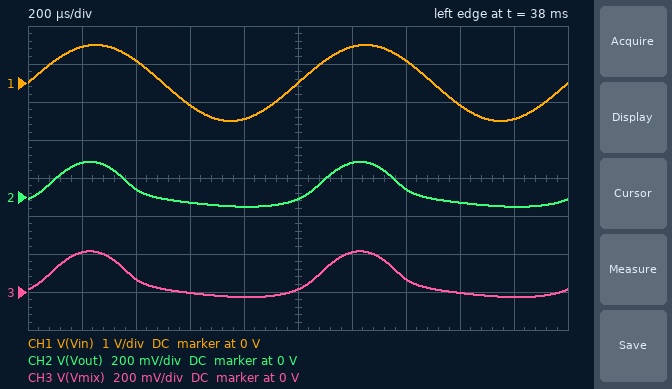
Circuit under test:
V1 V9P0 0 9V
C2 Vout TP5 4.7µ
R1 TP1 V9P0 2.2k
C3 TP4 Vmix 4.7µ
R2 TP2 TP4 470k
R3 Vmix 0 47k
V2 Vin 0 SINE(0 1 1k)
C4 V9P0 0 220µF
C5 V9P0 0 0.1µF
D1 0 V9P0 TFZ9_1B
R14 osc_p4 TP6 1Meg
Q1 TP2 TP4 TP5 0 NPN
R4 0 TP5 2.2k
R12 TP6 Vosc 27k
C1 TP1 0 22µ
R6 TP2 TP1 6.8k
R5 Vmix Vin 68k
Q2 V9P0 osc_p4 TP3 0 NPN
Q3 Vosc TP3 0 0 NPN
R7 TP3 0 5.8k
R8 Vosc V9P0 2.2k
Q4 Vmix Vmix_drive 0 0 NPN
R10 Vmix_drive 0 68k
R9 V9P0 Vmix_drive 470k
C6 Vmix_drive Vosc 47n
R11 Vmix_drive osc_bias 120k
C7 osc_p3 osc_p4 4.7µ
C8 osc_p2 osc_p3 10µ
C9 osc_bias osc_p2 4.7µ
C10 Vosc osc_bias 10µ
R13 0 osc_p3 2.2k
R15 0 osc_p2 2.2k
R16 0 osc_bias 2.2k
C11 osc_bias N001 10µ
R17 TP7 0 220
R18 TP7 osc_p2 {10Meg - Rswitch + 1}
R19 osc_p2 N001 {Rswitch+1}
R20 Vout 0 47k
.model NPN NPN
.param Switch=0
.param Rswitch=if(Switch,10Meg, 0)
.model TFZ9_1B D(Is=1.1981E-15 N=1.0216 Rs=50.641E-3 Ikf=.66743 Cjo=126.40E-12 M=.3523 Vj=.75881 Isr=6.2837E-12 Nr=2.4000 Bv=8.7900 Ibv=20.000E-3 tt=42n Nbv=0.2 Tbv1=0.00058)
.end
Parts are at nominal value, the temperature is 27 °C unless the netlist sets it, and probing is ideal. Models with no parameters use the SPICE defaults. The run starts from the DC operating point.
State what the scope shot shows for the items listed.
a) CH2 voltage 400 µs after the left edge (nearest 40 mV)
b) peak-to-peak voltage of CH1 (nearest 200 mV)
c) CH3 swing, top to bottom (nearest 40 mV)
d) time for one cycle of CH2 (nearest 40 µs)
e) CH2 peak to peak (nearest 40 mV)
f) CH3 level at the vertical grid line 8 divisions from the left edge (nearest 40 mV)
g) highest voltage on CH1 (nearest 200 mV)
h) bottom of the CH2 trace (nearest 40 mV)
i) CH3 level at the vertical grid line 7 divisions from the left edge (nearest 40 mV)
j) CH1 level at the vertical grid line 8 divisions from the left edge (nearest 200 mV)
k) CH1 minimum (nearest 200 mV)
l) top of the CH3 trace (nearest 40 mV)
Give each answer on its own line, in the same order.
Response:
40 mV
2.0 V
240 mV
1.00 ms
240 mV
0 V
1.0 V
-40 mV
80 mV
-600 mV
-1.0 V
200 mV
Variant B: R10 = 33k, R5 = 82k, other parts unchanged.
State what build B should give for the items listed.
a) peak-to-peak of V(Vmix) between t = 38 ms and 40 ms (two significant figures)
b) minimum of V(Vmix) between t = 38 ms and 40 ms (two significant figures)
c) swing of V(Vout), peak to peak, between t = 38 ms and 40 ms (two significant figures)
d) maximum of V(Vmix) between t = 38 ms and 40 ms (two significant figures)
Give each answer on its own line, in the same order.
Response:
420 mV
-160 mV
410 mV
260 mV
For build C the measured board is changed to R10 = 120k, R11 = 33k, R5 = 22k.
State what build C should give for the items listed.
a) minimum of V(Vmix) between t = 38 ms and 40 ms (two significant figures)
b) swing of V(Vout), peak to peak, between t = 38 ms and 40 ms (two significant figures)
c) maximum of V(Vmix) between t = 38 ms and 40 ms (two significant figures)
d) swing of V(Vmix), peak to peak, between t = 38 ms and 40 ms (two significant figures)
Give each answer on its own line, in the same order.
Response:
-260 mV
810 mV
570 mV
830 mV
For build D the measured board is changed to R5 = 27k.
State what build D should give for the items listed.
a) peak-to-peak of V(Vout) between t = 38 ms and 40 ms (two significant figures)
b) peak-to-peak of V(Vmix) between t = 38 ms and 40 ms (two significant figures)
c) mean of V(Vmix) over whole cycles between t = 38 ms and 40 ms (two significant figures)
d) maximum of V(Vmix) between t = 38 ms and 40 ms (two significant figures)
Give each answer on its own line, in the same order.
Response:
610 mV
620 mV
130 mV
510 mV
